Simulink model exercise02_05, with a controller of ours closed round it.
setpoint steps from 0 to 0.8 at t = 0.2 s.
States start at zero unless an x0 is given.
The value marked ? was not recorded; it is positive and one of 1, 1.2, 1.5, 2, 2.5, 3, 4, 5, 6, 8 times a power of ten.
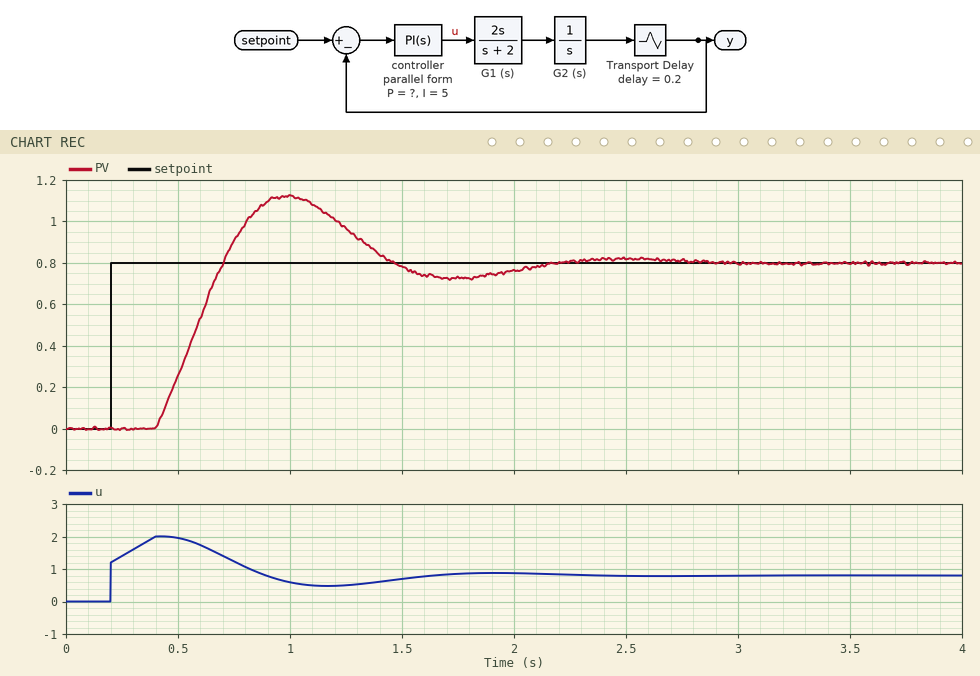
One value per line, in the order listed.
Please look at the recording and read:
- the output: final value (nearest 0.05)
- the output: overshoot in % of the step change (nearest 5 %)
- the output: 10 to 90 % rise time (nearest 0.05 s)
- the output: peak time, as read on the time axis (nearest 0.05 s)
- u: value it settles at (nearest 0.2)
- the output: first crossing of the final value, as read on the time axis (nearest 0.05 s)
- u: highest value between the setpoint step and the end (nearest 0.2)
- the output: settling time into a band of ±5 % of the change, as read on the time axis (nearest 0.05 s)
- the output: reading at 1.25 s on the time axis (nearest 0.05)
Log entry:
0.80
40 %
0.25 s
1.00 s
0.8
0.70 s
2.0
2.00 s
0.95
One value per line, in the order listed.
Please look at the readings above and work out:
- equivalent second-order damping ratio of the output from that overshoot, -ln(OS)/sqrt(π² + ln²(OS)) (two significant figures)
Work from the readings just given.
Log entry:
0.28
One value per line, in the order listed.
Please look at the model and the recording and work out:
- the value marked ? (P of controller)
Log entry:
1.5
